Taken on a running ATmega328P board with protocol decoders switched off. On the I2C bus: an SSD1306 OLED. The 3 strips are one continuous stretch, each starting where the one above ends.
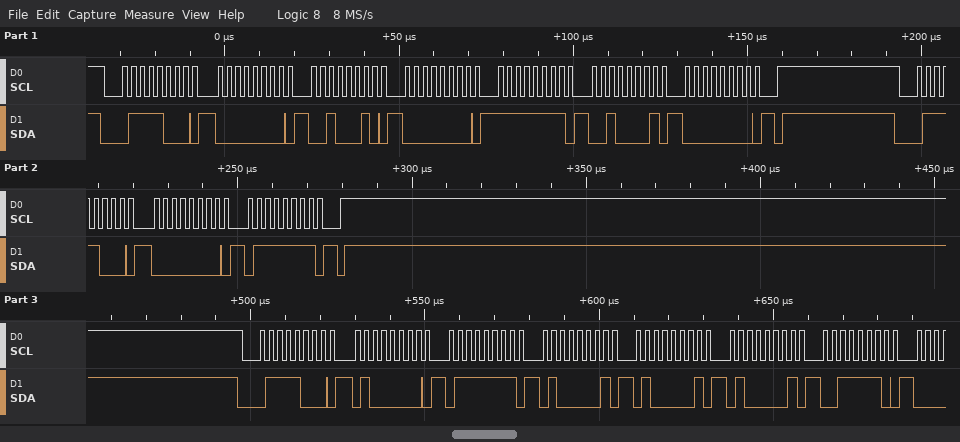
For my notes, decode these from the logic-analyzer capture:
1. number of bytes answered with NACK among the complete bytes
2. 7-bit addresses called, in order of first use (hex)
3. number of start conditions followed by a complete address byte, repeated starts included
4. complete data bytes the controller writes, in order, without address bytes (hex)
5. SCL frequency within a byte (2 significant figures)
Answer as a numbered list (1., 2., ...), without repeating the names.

1. 0
2. 0x3C
3. 3
4. 00 22 00 FF 21 00 00 7F 40 7F 41 41 41 3E
5. 400 kHz
